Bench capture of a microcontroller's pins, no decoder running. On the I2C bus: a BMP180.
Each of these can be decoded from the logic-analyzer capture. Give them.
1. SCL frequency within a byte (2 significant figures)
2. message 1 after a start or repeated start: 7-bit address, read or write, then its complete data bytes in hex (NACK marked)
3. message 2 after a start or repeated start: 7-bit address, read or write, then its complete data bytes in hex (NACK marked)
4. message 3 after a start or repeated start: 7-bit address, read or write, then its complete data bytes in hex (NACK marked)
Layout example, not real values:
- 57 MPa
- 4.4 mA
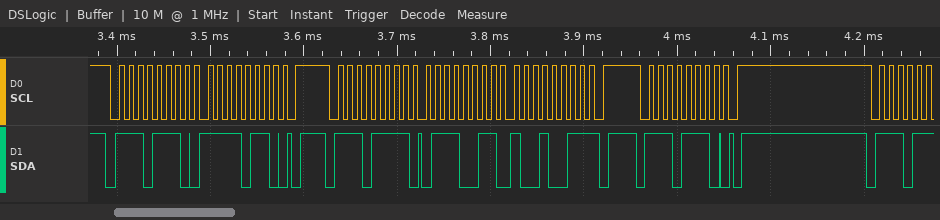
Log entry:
- 100 kHz
- 0x77 write: F6
- 0x77 read: 73 93 NACK
- 0x77 write
